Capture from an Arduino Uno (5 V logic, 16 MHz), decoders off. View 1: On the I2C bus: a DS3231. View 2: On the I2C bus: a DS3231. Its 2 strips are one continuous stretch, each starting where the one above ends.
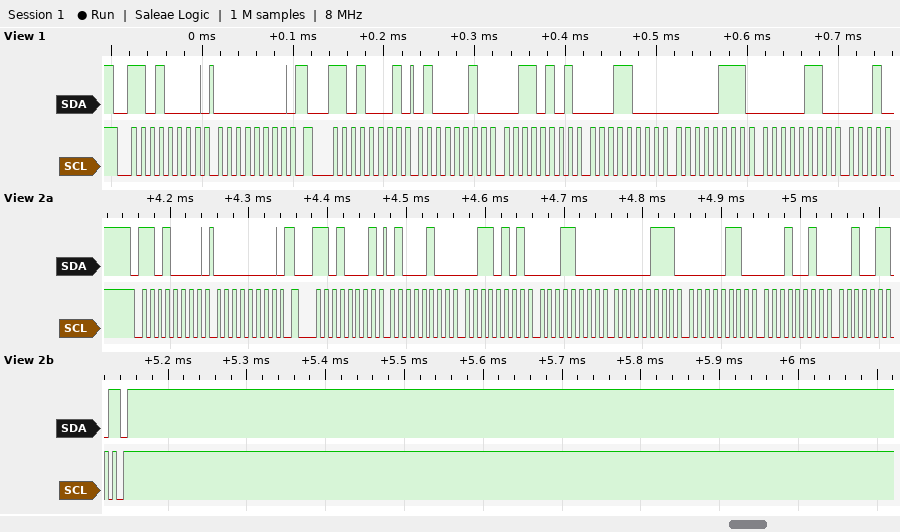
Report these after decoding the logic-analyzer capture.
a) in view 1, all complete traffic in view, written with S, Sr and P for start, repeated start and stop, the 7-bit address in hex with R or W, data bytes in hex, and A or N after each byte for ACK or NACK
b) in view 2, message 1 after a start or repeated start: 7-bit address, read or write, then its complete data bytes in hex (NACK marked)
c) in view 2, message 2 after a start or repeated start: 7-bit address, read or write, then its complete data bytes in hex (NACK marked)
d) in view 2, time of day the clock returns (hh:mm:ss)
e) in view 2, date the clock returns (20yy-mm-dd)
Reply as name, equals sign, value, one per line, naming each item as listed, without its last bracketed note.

in view 1, all complete traffic in view, written with S, Sr and P for start, repeated start and stop, the 7-bit address in hex with R or W, data bytes in hex, and A or N after each byte for ACK or NACK = S 68W A 00 A Sr 68R A 42 A 35 A 18 A 07 A 06 A
in view 2, message 1 after a start or repeated start: 7-bit address, read or write, then its complete data bytes in hex = 0x68 write: 00
in view 2, message 2 after a start or repeated start: 7-bit address, read or write, then its complete data bytes in hex = 0x68 read: 44 35 18 07 06 12 26 NACK
in view 2, time of day the clock returns = 18:35:44
in view 2, date the clock returns = 2026-12-06
